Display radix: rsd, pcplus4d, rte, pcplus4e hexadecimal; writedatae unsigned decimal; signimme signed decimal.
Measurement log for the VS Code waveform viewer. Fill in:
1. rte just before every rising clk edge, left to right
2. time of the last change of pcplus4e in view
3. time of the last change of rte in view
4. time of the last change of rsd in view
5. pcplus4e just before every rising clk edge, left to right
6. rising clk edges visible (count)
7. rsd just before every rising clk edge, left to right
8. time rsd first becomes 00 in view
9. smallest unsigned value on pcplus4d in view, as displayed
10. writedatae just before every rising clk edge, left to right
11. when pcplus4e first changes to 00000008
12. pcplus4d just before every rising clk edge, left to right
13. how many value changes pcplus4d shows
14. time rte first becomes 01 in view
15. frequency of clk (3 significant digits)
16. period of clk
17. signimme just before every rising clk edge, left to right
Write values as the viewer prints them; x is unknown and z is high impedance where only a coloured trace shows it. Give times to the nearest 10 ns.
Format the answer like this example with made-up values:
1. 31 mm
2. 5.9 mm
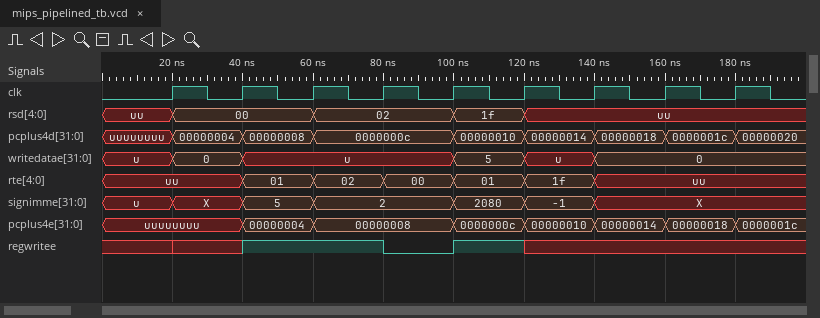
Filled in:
1. uu, uu, 01, 02, 00, 01, 1f, uu, uu
2. 180 ns
3. 140 ns
4. 120 ns
5. uuuuuuuu, uuuuuuuu, 00000004, 00000008, 00000008, 0000000c, 00000010, 00000014, 00000018
6. 9
7. uu, 00, 00, 02, 02, 1f, uu, uu, uu
8. 20 ns
9. 00000004
10. u, 0, u, u, u, 5, u, 0, 0
11. 60 ns
12. uuuuuuuu, 00000004, 00000008, 0000000c, 0000000c, 00000010, 00000014, 00000018, 0000001c
13. 8
14. 40 ns
15. 50.0 MHz
16. 20 ns
17. u, X, 5, 2, 2, 2080, -1, X, X
